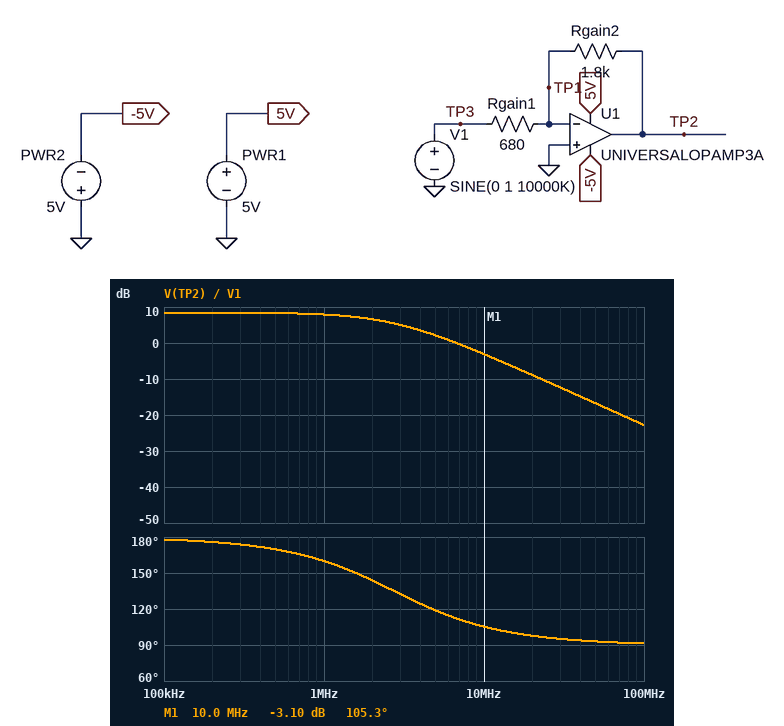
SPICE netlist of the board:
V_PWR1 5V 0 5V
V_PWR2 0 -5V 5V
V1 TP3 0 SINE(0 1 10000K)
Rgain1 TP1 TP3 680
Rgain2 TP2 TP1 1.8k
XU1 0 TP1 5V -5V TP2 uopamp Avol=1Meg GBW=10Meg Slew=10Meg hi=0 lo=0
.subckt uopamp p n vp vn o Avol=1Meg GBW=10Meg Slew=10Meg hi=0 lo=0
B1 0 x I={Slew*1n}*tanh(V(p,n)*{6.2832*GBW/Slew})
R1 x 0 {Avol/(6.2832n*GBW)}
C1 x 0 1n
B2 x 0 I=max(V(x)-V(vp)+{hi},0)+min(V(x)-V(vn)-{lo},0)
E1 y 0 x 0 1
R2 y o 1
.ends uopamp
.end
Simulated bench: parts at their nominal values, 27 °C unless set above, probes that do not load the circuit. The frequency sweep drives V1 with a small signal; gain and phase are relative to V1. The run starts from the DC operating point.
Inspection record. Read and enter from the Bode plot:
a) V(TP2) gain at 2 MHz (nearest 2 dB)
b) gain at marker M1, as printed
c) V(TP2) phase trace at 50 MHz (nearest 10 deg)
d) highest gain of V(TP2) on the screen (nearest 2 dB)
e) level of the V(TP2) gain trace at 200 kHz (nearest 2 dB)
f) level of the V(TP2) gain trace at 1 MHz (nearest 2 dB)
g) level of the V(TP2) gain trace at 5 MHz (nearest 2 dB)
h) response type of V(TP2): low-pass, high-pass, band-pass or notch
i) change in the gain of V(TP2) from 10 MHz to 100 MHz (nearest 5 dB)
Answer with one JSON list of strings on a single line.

["6 dB", "-3.10 dB", "90 deg", "8 dB", "8 dB", "8 dB", "2 dB", "low-pass", "-20 dB"]
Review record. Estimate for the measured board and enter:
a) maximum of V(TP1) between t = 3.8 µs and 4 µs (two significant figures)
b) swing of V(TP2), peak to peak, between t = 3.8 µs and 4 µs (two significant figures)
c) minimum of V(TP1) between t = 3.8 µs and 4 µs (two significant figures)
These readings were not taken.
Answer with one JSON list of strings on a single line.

["720 mV", "450 mV", "-720 mV"]
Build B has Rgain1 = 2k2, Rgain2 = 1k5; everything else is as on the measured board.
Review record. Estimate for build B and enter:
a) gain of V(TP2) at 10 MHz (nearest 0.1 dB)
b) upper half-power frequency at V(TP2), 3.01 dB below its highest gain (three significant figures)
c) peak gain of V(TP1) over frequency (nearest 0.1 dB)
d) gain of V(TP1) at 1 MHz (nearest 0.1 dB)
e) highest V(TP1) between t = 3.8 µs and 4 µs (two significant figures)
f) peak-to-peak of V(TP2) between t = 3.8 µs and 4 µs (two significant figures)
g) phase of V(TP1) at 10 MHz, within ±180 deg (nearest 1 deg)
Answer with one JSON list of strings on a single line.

["-9.2 dB", "5.94 MHz", "-7.8 dB", "-23.4 dB", "390 mV", "400 mV", "31 deg"]
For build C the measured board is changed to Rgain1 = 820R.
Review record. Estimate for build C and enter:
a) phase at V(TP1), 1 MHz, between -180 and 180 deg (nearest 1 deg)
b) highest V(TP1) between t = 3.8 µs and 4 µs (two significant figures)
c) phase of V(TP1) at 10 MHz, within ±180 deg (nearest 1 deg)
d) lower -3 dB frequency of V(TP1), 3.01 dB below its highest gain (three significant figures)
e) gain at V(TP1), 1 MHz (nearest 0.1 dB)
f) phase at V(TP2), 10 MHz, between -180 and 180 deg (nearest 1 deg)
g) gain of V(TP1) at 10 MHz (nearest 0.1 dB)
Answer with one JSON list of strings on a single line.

["72 deg", "680 mV", "17 deg", "3.13 MHz", "-13.6 dB", "107 deg", "-3.7 dB"]
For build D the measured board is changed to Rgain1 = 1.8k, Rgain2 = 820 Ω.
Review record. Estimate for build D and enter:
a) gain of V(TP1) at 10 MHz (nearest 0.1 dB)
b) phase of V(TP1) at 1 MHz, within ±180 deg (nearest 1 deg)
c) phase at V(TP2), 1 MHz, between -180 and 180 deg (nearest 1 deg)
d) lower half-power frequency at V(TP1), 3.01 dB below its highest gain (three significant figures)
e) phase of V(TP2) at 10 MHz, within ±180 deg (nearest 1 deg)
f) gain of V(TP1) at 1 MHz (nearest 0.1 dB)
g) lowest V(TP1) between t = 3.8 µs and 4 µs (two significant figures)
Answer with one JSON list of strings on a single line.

["-11.8 dB", "82 deg", "172 deg", "6.87 MHz", "124 deg", "-26.9 dB", "-290 mV"]
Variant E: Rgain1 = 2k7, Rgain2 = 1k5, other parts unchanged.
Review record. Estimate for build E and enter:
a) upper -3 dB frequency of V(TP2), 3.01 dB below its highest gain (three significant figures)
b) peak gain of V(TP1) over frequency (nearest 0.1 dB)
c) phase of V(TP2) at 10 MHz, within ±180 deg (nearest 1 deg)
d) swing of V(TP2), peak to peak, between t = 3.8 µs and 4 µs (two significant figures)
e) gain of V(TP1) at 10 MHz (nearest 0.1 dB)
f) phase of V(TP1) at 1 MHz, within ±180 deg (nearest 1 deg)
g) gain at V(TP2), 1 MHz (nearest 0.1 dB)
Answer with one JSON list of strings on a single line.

["6.43 MHz", "-8.9 dB", "123 deg", "390 mV", "-10.4 dB", "81 deg", "-5.2 dB"]
